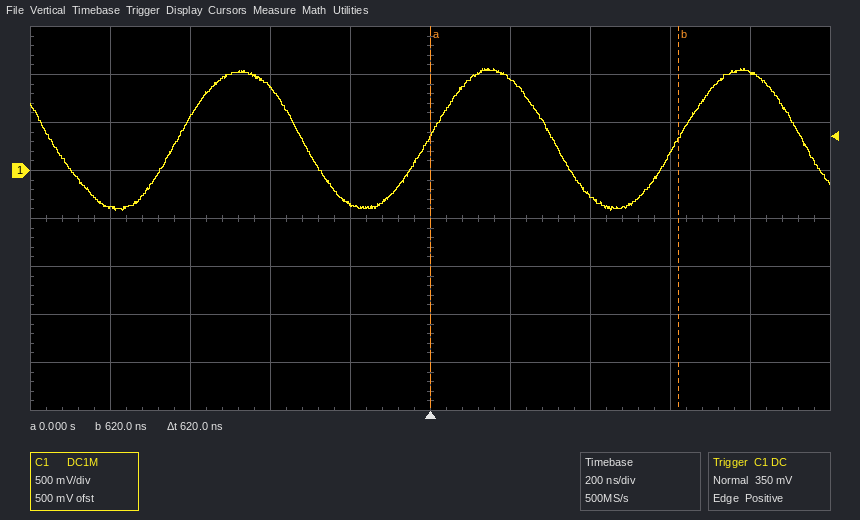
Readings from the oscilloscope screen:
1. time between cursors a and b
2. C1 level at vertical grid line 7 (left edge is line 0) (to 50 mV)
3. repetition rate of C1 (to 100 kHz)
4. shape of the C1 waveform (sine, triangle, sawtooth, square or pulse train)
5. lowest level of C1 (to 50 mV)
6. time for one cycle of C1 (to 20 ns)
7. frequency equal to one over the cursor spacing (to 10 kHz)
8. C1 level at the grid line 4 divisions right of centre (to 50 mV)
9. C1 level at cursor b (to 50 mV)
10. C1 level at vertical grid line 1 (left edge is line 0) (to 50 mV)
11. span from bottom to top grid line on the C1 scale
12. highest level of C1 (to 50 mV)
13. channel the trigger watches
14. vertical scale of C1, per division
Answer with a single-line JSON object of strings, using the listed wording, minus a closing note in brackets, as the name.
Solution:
{"time between cursors a and b": "620 ns", "C1 level at vertical grid line 7 (left edge is line 0)": "-250 mV", "repetition rate of C1": "1.6 MHz", "shape of the C1 waveform": "sine", "lowest level of C1": "-400 mV", "time for one cycle of C1": "620 ns", "frequency equal to one over the cursor spacing": "1.61 MHz", "C1 level at the grid line 4 divisions right of centre": "1.00 V", "C1 level at cursor b": "350 mV", "C1 level at vertical grid line 1 (left edge is line 0)": "-400 mV", "span from bottom to top grid line on the C1 scale": "4 V", "highest level of C1": "1.05 V", "channel the trigger watches": "C1", "vertical scale of C1, per division": "500 mV"}
